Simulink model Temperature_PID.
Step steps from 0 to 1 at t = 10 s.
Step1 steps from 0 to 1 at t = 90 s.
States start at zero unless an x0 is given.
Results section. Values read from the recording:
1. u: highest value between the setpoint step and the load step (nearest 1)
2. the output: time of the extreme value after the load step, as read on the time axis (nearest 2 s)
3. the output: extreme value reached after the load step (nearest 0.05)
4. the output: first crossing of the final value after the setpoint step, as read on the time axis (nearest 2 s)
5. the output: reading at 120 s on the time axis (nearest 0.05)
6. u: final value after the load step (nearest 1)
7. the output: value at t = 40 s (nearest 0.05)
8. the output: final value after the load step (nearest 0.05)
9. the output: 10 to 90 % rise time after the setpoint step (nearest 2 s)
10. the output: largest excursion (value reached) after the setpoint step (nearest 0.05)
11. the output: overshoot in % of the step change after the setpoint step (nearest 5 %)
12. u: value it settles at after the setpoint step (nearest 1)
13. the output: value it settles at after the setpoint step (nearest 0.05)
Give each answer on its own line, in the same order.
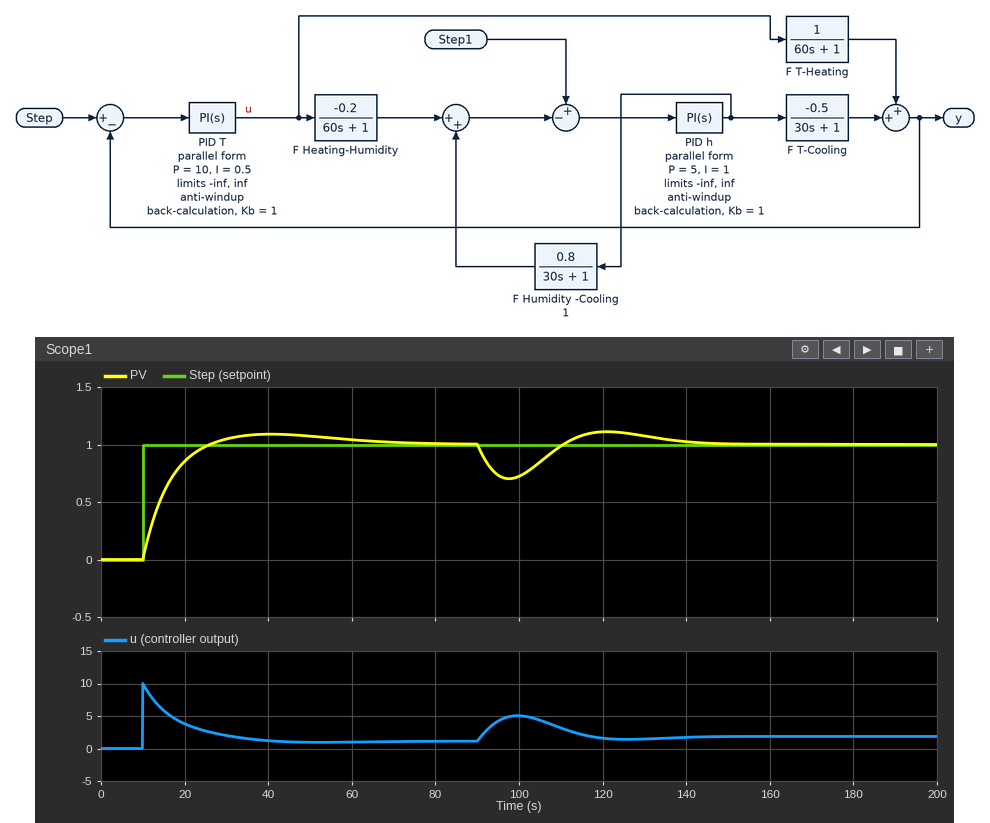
10
98 s
0.70
26 s
1.10
2
1.10
1.00
10 s
1.10
10 %
1
1.00
